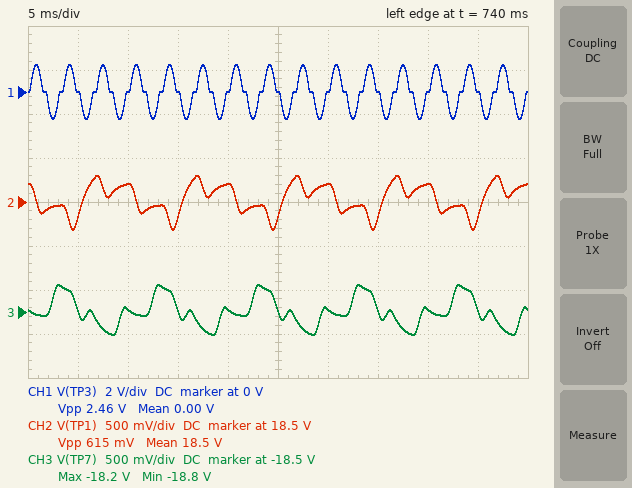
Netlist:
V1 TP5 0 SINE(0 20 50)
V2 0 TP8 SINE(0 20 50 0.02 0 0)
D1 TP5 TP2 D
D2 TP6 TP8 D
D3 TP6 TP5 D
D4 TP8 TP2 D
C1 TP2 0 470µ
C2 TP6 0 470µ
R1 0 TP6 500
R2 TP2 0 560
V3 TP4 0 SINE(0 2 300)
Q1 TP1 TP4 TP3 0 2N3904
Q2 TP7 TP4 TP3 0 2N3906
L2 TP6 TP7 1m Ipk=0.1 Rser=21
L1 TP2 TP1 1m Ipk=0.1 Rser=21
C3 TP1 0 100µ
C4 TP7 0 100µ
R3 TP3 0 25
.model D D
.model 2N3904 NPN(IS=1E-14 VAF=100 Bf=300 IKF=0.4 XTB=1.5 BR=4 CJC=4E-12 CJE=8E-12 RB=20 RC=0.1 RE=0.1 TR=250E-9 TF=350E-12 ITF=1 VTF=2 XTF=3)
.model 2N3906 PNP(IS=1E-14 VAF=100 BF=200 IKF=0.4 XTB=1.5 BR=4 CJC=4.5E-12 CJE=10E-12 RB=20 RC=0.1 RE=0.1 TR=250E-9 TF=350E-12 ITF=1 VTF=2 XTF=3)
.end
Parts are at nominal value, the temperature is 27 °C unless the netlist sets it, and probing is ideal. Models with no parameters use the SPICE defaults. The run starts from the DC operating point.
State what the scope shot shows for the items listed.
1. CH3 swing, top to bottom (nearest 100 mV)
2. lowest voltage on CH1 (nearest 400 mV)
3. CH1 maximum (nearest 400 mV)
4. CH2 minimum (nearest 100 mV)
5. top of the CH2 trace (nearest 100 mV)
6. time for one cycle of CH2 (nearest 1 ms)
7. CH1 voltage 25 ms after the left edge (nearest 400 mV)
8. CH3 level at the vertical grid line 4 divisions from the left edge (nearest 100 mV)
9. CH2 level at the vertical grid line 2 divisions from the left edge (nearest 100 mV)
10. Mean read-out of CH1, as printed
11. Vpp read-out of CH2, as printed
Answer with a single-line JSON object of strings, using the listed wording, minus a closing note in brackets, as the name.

{"CH3 swing, top to bottom": "600 mV", "lowest voltage on CH1": "-1.2 V", "CH1 maximum": "1.2 V", "CH2 minimum": "18.2 V", "top of the CH2 trace": "18.8 V", "time for one cycle of CH2": "10 ms", "CH1 voltage 25 ms after the left edge": "0 V", "CH3 level at the vertical grid line 4 divisions from the left edge": "-18.5 V", "CH2 level at the vertical grid line 2 divisions from the left edge": "18.7 V", "Mean read-out of CH1, as printed": "0.00 V", "Vpp read-out of CH2, as printed": "615 mV"}
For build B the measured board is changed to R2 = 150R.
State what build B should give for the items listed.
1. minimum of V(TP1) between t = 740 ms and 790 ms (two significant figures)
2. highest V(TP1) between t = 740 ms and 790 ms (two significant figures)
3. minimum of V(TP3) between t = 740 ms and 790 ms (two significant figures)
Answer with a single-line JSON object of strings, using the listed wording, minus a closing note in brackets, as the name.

{"minimum of V(TP1) between t = 740 ms and 790 ms": "17 V", "highest V(TP1) between t = 740 ms and 790 ms": "18 V", "minimum of V(TP3) between t = 740 ms and 790 ms": "-1.2 V"}
